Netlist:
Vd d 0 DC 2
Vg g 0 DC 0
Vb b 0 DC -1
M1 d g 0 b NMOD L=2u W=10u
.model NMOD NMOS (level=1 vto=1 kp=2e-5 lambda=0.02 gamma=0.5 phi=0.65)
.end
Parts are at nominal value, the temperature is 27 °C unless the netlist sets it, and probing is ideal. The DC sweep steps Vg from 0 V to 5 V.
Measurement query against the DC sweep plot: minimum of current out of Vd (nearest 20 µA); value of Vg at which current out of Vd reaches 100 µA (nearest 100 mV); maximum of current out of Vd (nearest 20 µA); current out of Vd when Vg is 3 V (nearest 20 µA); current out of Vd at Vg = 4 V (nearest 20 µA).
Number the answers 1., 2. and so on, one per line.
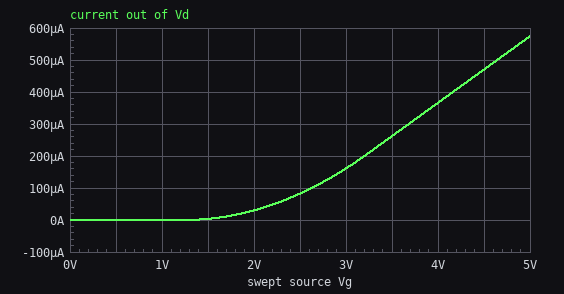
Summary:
1. 0 A
2. 2.6 V
3. 580 µA
4. 160 µA
5. 360 µA
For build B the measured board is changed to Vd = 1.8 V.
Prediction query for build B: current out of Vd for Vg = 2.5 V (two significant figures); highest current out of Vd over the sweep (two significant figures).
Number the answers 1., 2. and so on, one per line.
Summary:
1. 82 µA
2. 530 µA
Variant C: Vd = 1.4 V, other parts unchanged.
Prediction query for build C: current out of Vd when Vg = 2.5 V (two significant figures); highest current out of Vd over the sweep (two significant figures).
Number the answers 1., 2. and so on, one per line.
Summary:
1. 82 µA
2. 440 µA
